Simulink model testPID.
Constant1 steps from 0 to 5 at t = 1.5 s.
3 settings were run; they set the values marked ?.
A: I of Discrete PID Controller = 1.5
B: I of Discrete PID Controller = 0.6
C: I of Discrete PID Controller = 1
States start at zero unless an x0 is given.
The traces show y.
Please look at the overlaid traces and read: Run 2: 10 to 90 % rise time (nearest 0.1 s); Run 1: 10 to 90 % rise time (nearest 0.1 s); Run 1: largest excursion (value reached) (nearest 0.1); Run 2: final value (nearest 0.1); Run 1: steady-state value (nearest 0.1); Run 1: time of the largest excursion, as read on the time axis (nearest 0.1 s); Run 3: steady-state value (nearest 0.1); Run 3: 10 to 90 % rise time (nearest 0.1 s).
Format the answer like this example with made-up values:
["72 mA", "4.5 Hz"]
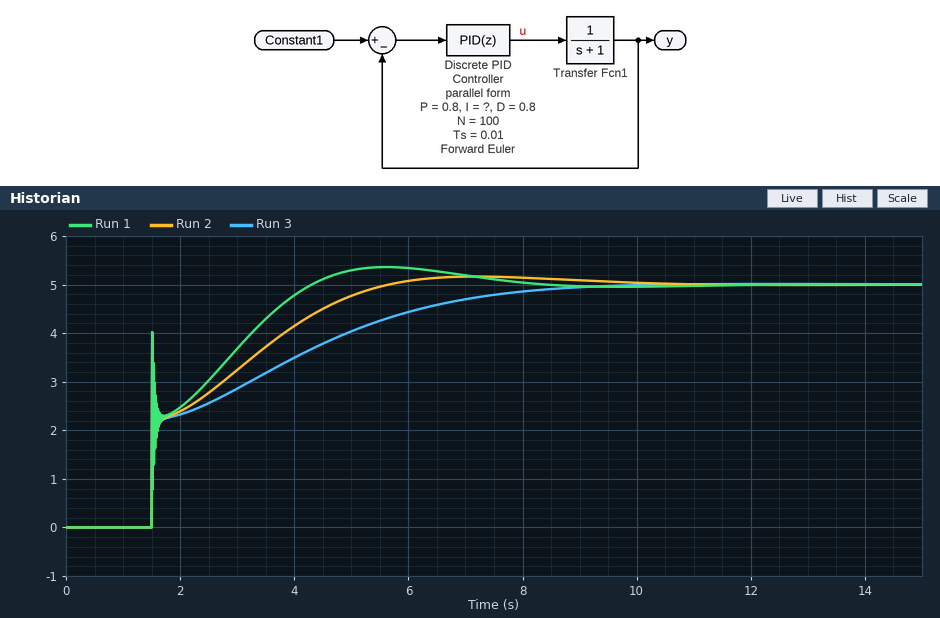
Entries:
["3.0 s", "2.2 s", "5.4", "5.0", "5.0", "5.6 s", "5.0", "4.7 s"]
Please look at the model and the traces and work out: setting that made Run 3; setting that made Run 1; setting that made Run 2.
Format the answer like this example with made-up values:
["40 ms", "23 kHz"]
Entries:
["B", "A", "C"]
